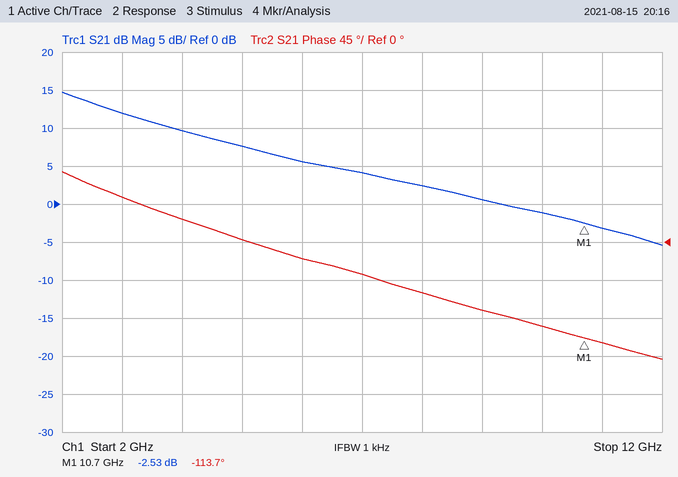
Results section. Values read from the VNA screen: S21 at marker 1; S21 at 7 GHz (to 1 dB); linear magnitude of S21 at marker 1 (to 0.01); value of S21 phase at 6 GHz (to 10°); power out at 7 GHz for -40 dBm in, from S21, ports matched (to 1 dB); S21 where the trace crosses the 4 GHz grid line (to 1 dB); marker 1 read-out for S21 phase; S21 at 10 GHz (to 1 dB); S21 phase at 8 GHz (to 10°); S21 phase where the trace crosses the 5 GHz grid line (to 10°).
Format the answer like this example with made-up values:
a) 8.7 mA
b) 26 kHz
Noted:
a) -2.53 dB
b) 4 dB
c) 0.75
d) -20°
e) -36 dBm
f) 10 dB
g) -113.7°
h) -1 dB
i) -60°
j) 0°
